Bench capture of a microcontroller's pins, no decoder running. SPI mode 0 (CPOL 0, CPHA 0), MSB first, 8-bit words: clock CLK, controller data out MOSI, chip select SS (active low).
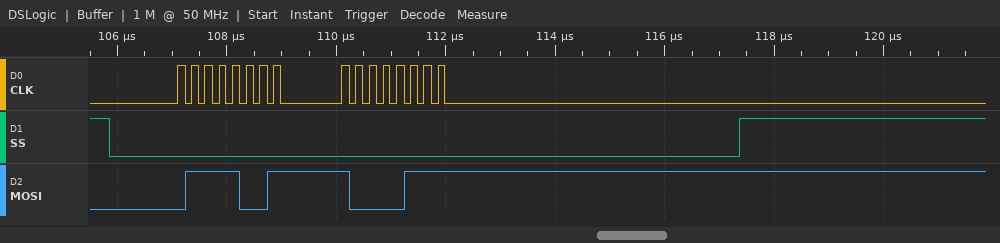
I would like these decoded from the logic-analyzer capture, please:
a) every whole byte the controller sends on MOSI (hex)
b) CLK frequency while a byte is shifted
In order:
79 87
4 MHz
